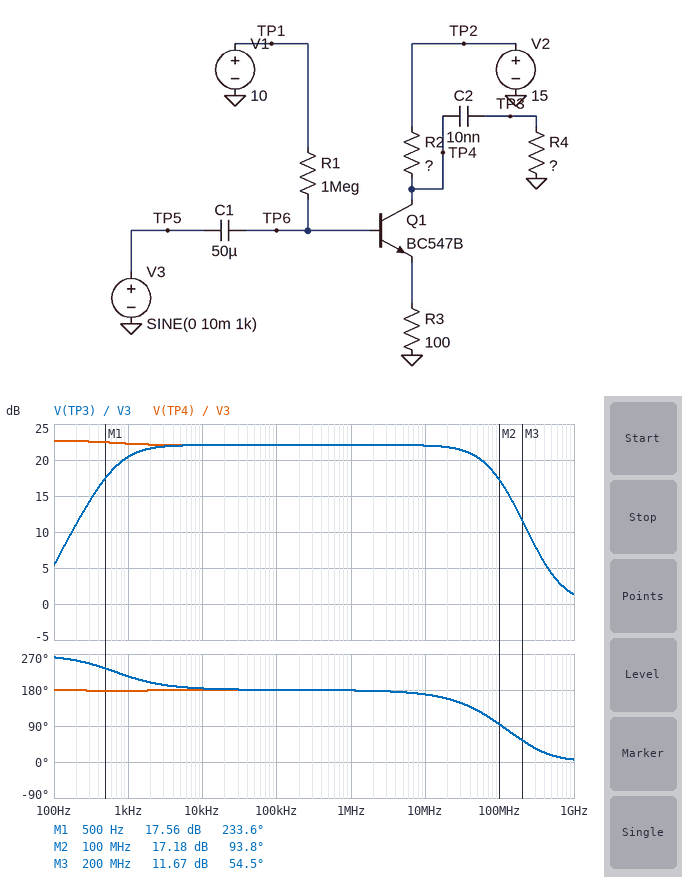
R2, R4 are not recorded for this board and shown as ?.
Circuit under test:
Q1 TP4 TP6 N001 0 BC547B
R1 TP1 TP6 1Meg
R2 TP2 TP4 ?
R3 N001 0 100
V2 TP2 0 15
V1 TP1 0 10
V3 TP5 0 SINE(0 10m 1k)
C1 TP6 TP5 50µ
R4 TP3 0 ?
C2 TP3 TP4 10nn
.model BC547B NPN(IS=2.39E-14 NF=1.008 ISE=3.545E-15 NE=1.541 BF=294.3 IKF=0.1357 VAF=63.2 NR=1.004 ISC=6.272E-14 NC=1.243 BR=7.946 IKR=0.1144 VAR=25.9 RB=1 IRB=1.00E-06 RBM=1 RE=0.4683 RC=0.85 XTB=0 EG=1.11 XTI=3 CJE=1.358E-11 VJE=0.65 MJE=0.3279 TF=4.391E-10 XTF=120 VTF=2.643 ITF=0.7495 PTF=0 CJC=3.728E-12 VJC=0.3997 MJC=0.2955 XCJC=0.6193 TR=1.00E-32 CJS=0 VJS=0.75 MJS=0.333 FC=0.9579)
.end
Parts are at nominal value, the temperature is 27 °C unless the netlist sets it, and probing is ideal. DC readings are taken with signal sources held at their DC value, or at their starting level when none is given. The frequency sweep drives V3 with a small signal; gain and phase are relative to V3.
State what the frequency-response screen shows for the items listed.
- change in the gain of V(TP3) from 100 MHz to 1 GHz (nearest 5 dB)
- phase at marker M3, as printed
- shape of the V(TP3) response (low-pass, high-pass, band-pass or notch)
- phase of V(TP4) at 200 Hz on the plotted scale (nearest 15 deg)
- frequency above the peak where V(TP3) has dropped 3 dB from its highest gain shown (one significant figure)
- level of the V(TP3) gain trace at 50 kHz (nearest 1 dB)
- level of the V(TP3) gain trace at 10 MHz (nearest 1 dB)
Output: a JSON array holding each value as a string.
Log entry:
["-15 dB", "54.5 deg", "band-pass", "180 deg", "70 MHz", "22 dB", "22 dB"]
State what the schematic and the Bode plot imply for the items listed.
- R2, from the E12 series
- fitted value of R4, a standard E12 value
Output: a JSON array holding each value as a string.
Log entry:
["1.5 kΩ", "22 kΩ"]
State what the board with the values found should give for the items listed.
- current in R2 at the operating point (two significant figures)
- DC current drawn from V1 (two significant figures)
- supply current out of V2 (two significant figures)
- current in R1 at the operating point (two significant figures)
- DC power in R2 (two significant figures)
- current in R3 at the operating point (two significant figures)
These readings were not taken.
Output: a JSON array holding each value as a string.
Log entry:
["2.9 mA", "9.0 µA", "2.9 mA", "9.0 µA", "13 mW", "2.9 mA"]
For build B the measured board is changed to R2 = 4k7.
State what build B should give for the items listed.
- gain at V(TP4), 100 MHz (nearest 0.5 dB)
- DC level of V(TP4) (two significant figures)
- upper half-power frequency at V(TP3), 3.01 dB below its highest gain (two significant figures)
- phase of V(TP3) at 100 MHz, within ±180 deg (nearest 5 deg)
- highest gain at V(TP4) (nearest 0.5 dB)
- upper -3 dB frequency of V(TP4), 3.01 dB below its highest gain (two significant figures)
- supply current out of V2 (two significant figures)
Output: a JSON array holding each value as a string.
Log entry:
["15.5 dB", "2.7 V", "18 MHz", "60 deg", "32.5 dB", "11 MHz", "2.6 mA"]
